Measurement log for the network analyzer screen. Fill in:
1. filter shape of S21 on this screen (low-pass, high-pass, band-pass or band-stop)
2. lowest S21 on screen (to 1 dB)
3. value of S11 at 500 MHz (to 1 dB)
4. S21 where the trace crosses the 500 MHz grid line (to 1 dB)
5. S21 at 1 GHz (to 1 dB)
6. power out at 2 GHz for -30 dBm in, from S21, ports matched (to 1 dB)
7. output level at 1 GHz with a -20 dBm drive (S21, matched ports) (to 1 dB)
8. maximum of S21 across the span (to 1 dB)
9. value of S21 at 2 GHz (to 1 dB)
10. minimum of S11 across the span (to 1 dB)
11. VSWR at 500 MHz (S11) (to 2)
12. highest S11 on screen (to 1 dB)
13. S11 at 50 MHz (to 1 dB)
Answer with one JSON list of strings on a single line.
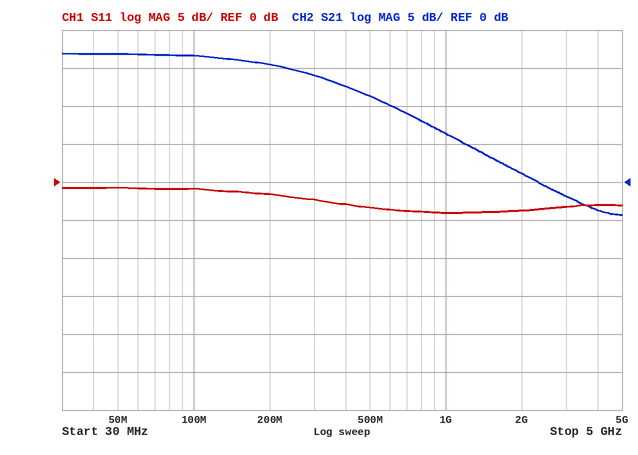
["low-pass", "-4 dB", "-3 dB", "11 dB", "6 dB", "-29 dBm", "-14 dBm", "17 dB", "1 dB", "-4 dB", "6", "-1 dB", "-1 dB"]
